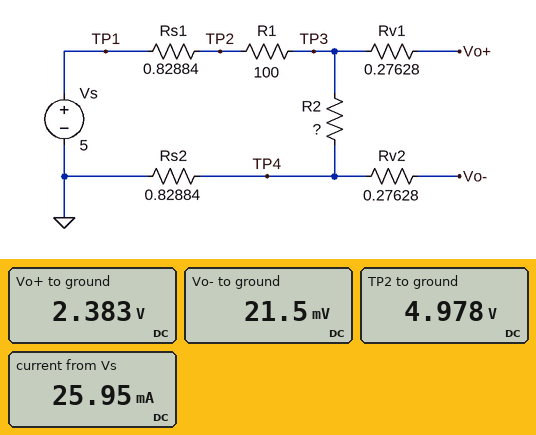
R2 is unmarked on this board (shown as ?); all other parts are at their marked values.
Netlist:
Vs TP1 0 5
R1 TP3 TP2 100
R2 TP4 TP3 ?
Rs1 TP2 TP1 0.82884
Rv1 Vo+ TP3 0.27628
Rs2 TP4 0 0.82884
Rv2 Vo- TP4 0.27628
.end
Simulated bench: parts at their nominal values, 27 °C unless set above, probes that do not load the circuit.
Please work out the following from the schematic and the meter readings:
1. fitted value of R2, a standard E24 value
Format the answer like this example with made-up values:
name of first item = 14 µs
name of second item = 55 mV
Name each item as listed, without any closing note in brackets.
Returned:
fitted value of R2, a standard E24 value = 91 Ω
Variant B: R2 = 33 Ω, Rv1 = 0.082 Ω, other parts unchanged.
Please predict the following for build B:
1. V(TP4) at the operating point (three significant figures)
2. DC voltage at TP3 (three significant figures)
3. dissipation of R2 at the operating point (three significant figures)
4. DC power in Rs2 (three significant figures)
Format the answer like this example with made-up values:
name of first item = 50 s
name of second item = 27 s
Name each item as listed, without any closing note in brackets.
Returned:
V(TP4) at the operating point = 30.8 mV
DC voltage at TP3 = 1.26 V
dissipation of R2 at the operating point = 45.5 mW
DC power in Rs2 = 1.14 mW
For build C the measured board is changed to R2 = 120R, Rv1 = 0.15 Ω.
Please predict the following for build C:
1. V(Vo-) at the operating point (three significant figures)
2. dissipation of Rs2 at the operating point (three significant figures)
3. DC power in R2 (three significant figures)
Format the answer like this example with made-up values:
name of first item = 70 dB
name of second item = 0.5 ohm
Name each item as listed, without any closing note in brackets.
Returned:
V(Vo-) at the operating point = 18.7 mV
dissipation of Rs2 at the operating point = 422 µW
DC power in R2 = 61.1 mW
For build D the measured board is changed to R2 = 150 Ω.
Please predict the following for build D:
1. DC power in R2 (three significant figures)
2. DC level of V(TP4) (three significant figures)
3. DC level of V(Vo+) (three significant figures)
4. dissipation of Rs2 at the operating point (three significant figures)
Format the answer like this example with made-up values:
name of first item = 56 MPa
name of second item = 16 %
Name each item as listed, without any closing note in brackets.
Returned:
DC power in R2 = 59.2 mW
DC level of V(TP4) = 16.5 mV
DC level of V(Vo+) = 3.00 V
dissipation of Rs2 at the operating point = 327 µW
